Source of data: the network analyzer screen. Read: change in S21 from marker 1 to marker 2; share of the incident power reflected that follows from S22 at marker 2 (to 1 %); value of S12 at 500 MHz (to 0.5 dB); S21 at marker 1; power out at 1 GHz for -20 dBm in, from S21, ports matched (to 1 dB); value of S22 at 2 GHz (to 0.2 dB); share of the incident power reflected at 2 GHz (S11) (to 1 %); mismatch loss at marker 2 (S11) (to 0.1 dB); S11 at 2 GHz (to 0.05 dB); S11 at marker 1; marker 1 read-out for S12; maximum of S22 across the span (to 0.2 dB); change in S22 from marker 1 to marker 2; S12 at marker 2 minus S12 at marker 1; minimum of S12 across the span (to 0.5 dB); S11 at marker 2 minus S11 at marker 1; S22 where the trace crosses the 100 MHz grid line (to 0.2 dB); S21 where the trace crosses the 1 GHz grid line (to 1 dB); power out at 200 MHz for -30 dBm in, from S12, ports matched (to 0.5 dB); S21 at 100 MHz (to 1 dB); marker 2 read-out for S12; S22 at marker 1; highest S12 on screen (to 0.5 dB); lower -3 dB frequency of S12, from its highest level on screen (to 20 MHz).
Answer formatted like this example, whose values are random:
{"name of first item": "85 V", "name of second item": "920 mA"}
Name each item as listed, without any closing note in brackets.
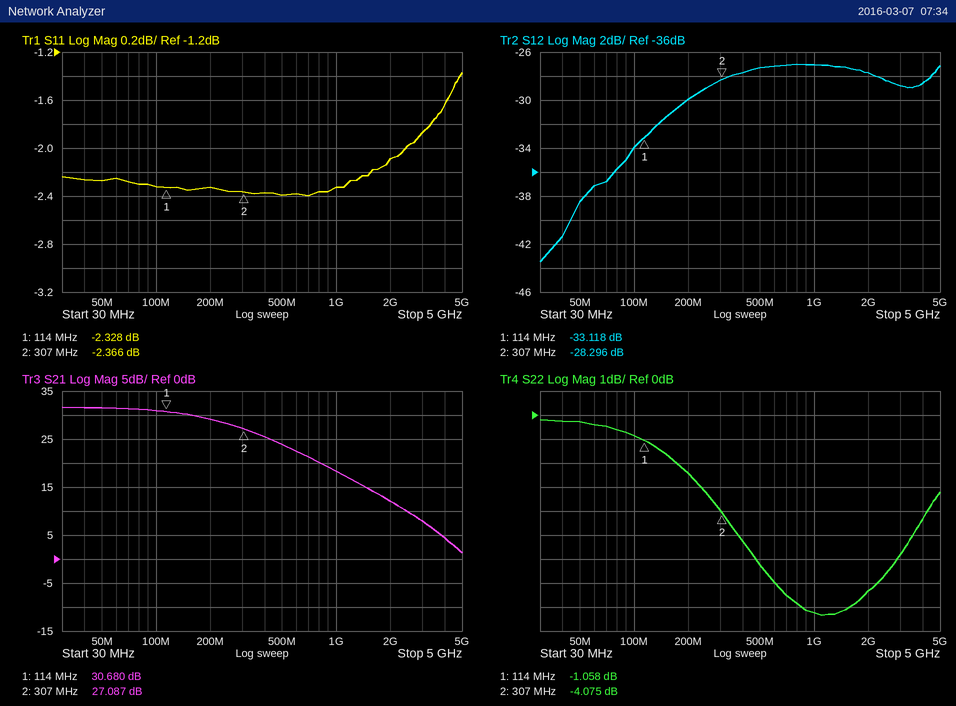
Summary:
{"change in S21 from marker 1 to marker 2": "-3.593 dB", "share of the incident power reflected that follows from S22 at marker 2": "39 %", "value of S12 at 500 MHz": "-27.5 dB", "S21 at marker 1": "30.680 dB", "power out at 1 GHz for -20 dBm in, from S21, ports matched": "-2 dBm", "value of S22 at 2 GHz": "-7.4 dB", "share of the incident power reflected at 2 GHz (S11)": "62 %", "mismatch loss at marker 2 (S11)": "3.8 dB", "S11 at 2 GHz": "-2.10 dB", "S11 at marker 1": "-2.328 dB", "marker 1 read-out for S12": "-33.118 dB", "maximum of S22 across the span": "-0.2 dB", "change in S22 from marker 1 to marker 2": "-3.017 dB", "S12 at marker 2 minus S12 at marker 1": "4.822 dB", "minimum of S12 across the span": "-43.5 dB", "S11 at marker 2 minus S11 at marker 1": "-0.038 dB", "S22 where the trace crosses the 100 MHz grid line": "-0.8 dB", "S21 where the trace crosses the 1 GHz grid line": "18 dB", "power out at 200 MHz for -30 dBm in, from S12, ports matched": "-60.0 dBm", "S21 at 100 MHz": "31 dB", "marker 2 read-out for S12": "-28.296 dB", "S22 at marker 1": "-1.058 dB", "highest S12 on screen": "-27.0 dB", "lower -3 dB frequency of S12, from its highest level on screen": "200 MHz"}
